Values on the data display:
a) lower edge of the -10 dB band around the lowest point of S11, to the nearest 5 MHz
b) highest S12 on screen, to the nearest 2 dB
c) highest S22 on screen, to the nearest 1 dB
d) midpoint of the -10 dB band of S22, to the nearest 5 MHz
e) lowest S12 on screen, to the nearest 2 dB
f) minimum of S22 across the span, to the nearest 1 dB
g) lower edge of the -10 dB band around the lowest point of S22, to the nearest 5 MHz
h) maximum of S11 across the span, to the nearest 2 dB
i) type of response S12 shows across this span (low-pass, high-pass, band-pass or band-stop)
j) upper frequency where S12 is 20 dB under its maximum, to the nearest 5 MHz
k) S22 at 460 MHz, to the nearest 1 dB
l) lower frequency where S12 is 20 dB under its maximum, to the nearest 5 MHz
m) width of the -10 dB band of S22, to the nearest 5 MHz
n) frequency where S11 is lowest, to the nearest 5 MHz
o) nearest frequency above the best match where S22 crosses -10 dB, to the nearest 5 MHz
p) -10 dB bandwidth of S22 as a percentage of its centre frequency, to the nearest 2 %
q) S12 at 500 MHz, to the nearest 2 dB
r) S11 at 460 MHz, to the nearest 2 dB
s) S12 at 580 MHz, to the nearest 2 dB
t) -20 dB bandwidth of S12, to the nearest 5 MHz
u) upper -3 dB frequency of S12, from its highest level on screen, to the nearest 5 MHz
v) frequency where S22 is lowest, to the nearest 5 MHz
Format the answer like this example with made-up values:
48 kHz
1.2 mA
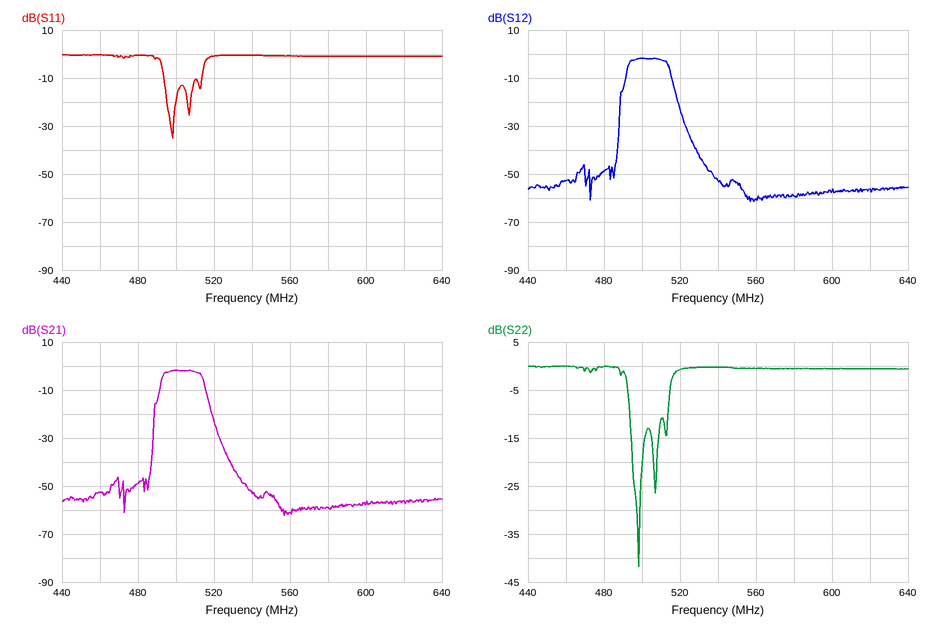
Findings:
495 MHz
-2 dB
0 dB
505 MHz
-62 dB
-42 dB
495 MHz
0 dB
band-pass
520 MHz
0 dB
490 MHz
20 MHz
500 MHz
515 MHz
4 %
-2 dB
0 dB
-60 dB
30 MHz
515 MHz
500 MHz
